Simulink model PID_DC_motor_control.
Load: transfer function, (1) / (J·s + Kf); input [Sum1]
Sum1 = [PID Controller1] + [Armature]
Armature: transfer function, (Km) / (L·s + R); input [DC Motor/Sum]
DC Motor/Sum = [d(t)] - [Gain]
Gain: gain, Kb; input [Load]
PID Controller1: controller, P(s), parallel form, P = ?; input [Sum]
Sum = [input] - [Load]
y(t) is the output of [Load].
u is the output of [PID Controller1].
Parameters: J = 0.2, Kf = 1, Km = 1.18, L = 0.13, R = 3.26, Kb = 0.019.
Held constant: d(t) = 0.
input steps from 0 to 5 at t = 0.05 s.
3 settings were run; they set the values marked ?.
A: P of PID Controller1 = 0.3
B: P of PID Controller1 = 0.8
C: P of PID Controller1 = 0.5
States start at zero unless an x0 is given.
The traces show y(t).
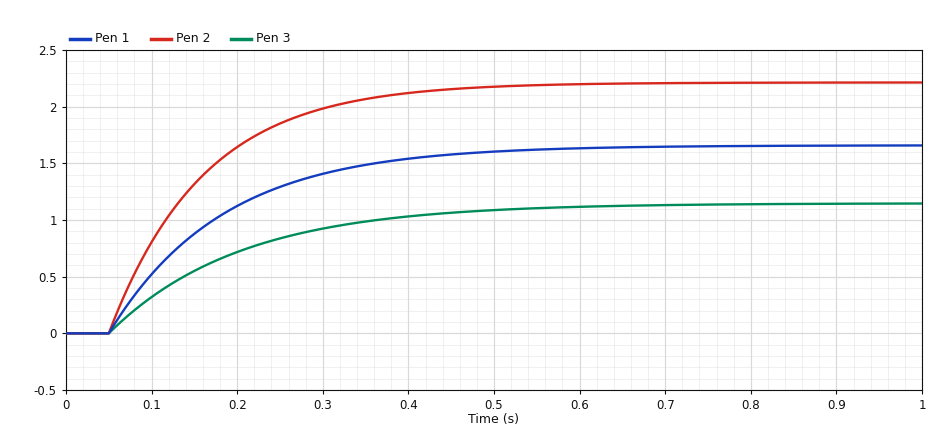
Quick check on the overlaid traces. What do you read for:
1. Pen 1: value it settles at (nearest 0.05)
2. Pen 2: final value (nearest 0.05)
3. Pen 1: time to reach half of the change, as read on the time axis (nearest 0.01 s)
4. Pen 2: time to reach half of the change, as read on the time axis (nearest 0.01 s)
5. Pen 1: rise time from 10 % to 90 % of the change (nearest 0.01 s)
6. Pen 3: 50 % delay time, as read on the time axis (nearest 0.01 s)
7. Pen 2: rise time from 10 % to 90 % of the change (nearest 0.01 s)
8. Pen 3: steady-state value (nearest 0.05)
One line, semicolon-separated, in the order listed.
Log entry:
1.65; 2.20; 0.14 s; 0.13 s; 0.29 s; 0.16 s; 0.24 s; 1.15
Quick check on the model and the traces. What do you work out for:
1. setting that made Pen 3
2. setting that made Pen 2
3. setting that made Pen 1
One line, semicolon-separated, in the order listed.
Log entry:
A; B; C
